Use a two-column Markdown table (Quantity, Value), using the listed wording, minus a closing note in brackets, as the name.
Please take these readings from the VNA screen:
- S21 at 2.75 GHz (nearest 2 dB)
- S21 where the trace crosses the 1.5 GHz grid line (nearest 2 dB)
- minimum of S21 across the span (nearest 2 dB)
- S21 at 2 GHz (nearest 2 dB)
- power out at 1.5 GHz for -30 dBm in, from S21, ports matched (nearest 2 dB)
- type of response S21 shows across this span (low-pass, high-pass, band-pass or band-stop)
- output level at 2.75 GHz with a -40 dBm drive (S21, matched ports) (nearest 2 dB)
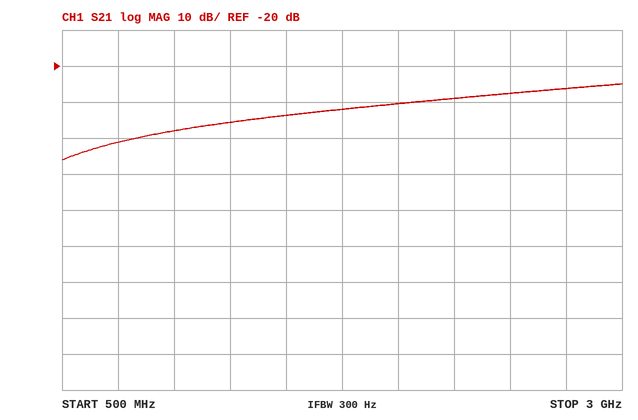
| Quantity | Value |
|---|---|
| S21 at 2.75 GHz | -26 dB |
| S21 where the trace crosses the 1.5 GHz grid line | -34 dB |
| minimum of S21 across the span | -46 dB |
| S21 at 2 GHz | -30 dB |
| power out at 1.5 GHz for -30 dBm in, from S21, ports matched | -64 dBm |
| type of response S21 shows across this span | high-pass |
| output level at 2.75 GHz with a -40 dBm drive (S21, matched ports) | -66 dBm |
